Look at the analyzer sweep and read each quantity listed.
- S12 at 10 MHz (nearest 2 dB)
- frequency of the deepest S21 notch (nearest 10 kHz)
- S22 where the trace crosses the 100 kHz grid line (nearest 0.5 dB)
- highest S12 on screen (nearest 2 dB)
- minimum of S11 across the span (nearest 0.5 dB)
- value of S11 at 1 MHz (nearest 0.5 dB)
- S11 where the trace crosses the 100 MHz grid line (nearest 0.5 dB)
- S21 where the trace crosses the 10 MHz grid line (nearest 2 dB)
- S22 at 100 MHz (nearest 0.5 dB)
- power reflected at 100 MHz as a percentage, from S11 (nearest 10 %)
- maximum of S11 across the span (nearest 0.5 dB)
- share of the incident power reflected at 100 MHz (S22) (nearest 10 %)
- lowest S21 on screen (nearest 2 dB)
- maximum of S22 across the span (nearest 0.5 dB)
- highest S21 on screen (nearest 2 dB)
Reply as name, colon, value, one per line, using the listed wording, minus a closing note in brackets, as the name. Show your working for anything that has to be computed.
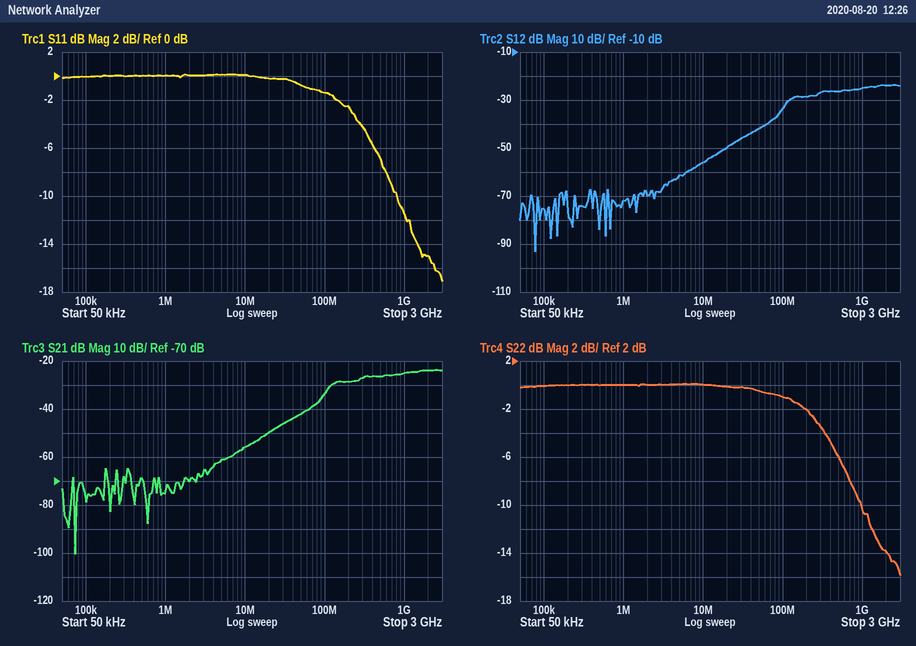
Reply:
S12 at 10 MHz: -56 dB
frequency of the deepest S21 notch: 70 kHz
S22 where the trace crosses the 100 kHz grid line: 0.0 dB
highest S12 on screen: -24 dB
minimum of S11 across the span: -17.0 dB
value of S11 at 1 MHz: 0.0 dB
S11 where the trace crosses the 100 MHz grid line: -1.5 dB
S21 where the trace crosses the 10 MHz grid line: -56 dB
S22 at 100 MHz: -1.0 dB
power reflected at 100 MHz as a percentage, from S11: 10^(-1.5/10) ≈ 70.8 %, so 70 % to the nearest 10 %
maximum of S11 across the span: 0.0 dB
share of the incident power reflected at 100 MHz (S22): 10^(-1/10) ≈ 79.4 %, so 80 % to the nearest 10 %
lowest S21 on screen: -100 dB
maximum of S22 across the span: 0.0 dB
highest S21 on screen: -24 dB
